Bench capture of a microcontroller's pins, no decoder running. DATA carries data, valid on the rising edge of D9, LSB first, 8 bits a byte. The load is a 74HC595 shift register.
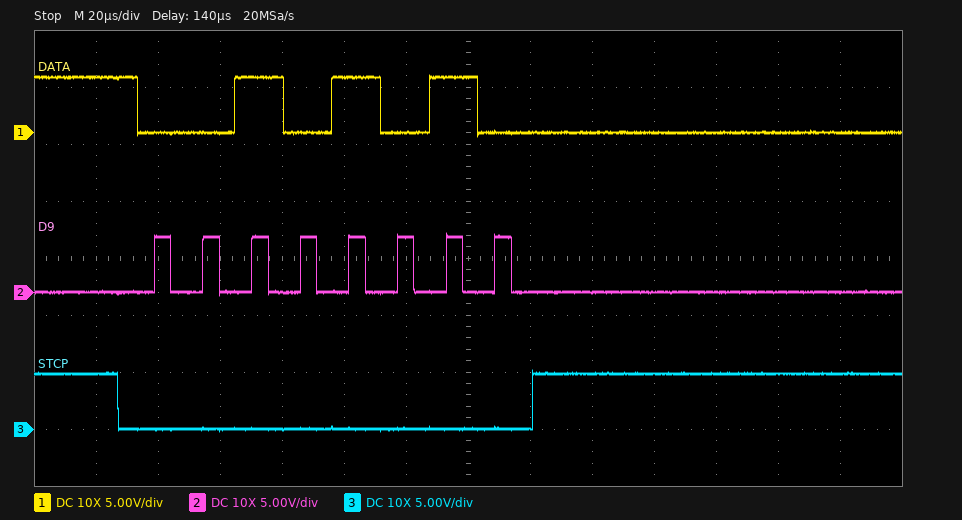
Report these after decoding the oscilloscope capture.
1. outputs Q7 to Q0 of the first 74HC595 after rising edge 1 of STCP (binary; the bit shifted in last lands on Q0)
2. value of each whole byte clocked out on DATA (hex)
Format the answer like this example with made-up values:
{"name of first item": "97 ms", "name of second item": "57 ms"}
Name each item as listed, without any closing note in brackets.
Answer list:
{"outputs Q7 to Q0 of the first 74HC595 after rising edge 1 of STCP": "00101010", "value of each whole byte clocked out on DATA": "54"}
